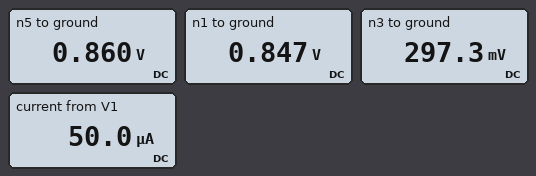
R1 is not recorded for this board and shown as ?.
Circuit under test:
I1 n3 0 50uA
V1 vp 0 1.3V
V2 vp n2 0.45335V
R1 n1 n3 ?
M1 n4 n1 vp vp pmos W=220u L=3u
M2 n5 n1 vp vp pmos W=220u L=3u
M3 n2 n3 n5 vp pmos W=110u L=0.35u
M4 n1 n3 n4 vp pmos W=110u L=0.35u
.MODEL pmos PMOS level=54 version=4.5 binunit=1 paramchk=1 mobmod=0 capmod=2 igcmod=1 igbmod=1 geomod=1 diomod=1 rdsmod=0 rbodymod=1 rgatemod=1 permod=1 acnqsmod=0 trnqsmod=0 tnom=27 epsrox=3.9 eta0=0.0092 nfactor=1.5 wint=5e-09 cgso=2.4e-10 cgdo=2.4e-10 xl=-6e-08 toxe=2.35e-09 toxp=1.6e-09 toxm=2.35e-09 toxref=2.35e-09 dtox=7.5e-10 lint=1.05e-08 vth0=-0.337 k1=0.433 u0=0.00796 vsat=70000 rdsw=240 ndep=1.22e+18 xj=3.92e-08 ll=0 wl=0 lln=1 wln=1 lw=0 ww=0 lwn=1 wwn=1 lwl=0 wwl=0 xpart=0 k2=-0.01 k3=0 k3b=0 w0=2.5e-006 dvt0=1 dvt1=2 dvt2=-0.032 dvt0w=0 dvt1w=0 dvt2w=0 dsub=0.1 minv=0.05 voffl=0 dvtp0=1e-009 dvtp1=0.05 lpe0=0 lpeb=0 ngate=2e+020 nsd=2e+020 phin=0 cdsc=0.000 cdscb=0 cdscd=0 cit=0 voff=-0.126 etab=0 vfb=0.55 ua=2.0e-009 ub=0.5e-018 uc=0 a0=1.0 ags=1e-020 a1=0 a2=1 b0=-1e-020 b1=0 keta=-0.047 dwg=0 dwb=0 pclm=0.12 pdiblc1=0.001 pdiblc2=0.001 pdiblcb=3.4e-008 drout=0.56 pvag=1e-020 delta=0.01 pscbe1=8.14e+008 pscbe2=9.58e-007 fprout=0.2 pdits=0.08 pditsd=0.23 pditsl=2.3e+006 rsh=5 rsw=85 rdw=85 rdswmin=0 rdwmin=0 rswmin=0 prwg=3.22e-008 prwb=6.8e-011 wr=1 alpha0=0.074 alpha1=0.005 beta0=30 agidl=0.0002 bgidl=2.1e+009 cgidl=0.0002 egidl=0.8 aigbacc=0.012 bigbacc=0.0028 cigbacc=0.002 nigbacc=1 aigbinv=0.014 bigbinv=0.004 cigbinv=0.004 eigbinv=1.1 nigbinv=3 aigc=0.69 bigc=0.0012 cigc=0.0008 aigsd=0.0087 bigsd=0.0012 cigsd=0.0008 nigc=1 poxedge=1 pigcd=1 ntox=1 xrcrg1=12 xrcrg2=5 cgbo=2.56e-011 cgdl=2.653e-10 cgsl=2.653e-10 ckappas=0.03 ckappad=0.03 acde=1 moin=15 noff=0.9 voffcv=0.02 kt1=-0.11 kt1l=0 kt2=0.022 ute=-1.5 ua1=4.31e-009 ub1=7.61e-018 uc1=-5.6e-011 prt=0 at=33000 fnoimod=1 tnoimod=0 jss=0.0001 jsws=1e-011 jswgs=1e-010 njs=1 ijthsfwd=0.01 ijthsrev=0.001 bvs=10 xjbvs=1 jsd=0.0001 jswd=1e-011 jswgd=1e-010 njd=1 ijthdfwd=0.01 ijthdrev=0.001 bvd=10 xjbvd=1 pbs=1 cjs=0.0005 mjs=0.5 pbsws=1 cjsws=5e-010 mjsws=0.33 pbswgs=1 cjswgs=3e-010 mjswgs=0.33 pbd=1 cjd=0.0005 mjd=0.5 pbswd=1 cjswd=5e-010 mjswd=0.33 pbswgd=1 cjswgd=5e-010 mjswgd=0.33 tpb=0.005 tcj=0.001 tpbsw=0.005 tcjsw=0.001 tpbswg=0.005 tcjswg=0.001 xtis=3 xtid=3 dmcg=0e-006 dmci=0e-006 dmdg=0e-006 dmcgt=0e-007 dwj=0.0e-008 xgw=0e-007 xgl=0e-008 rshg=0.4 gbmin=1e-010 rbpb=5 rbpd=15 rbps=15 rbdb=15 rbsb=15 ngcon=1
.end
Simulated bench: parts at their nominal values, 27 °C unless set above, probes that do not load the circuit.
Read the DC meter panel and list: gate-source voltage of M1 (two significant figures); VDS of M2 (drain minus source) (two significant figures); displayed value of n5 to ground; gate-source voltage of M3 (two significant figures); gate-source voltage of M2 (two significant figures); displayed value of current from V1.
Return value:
-450 mV
-440 mV
0.860 V
-560 mV
-450 mV
50.0 µA
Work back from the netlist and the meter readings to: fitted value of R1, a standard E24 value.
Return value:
11 kΩ
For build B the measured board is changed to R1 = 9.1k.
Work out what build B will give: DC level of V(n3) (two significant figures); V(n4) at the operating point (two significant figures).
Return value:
390 mV
880 mV
